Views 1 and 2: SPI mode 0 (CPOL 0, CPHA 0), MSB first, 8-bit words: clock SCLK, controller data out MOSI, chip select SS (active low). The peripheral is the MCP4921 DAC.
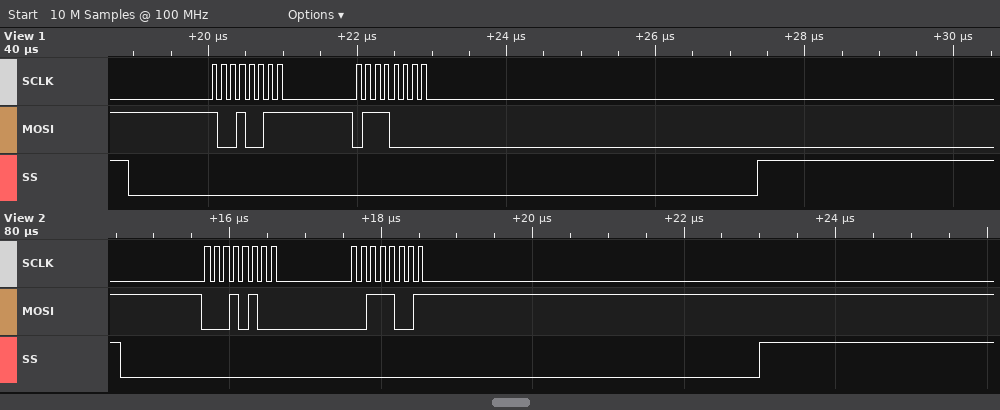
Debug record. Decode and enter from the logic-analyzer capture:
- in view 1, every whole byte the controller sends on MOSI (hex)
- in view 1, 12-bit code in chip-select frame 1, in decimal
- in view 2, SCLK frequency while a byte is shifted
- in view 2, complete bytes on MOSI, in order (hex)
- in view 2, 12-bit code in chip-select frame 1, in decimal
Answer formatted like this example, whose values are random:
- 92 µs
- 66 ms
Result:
- 93 70
- 880
- 8 MHz
- 14 39
- 1081
